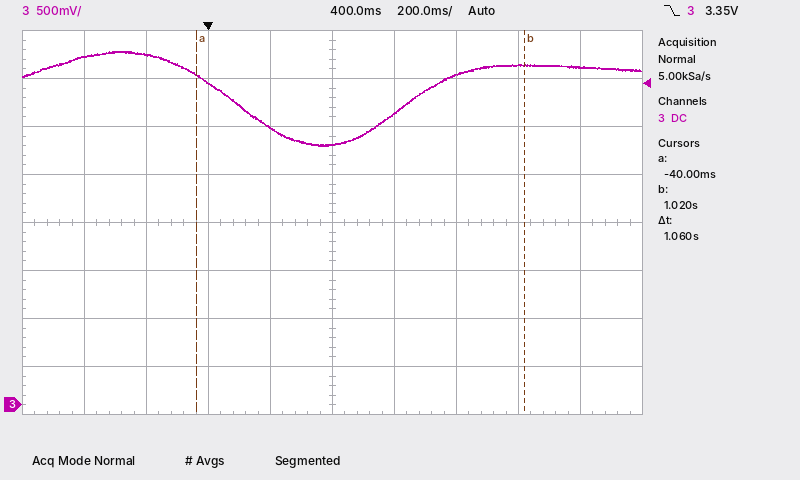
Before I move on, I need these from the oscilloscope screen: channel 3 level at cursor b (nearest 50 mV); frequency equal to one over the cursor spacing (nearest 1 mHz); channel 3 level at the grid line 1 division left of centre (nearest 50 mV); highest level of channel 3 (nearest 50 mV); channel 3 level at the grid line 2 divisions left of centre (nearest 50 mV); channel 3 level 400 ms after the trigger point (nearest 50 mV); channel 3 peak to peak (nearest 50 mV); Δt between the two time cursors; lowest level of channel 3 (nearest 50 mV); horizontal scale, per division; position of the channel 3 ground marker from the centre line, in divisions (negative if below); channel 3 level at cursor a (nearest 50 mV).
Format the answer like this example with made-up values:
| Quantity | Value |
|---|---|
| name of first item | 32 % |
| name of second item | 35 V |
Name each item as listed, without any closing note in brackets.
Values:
| Quantity | Value |
|---|---|
| channel 3 level at cursor b | 3.55 V |
| frequency equal to one over the cursor spacing | 943 mHz |
| channel 3 level at the grid line 1 division left of centre | 2.90 V |
| highest level of channel 3 | 3.70 V |
| channel 3 level at the grid line 2 divisions left of centre | 3.35 V |
| channel 3 level 400 ms after the trigger point | 2.70 V |
| channel 3 peak to peak | 1.00 V |
| Δt between the two time cursors | 1.06 s |
| lowest level of channel 3 | 2.70 V |
| horizontal scale, per division | 200 ms |
| position of the channel 3 ground marker from the centre line, in divisions | -3.8 div |
| channel 3 level at cursor a | 3.45 V |
